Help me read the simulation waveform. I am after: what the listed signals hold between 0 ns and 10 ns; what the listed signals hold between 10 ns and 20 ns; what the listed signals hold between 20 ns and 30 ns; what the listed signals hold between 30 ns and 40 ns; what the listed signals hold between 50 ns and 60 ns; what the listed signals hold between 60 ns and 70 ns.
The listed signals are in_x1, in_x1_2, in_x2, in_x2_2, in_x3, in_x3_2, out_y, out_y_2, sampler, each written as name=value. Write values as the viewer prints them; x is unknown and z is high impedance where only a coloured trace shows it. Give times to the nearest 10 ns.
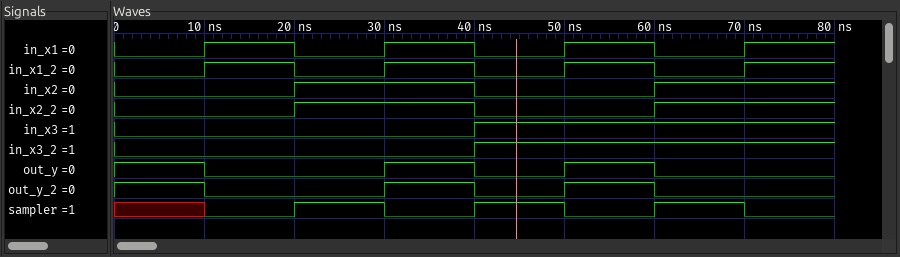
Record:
in_x1=0, in_x1_2=0, in_x2=0, in_x2_2=0, in_x3=0, in_x3_2=0, out_y=1, out_y_2=1, sampler=x
in_x1=1, in_x1_2=1, in_x2=0, in_x2_2=0, in_x3=0, in_x3_2=0, out_y=0, out_y_2=0, sampler=0
in_x1=0, in_x1_2=0, in_x2=1, in_x2_2=1, in_x3=0, in_x3_2=0, out_y=0, out_y_2=0, sampler=1
in_x1=1, in_x1_2=1, in_x2=1, in_x2_2=1, in_x3=0, in_x3_2=0, out_y=1, out_y_2=1, sampler=0
in_x1=1, in_x1_2=1, in_x2=0, in_x2_2=0, in_x3=1, in_x3_2=1, out_y=1, out_y_2=1, sampler=0
in_x1=0, in_x1_2=0, in_x2=1, in_x2_2=1, in_x3=1, in_x3_2=1, out_y=0, out_y_2=0, sampler=1
